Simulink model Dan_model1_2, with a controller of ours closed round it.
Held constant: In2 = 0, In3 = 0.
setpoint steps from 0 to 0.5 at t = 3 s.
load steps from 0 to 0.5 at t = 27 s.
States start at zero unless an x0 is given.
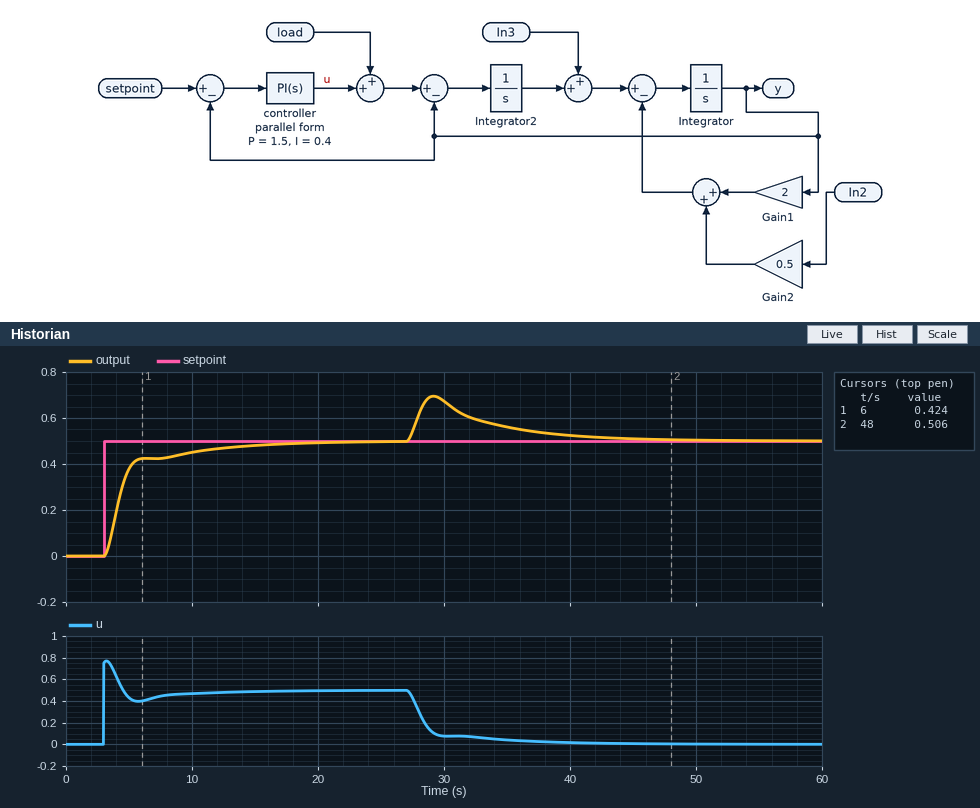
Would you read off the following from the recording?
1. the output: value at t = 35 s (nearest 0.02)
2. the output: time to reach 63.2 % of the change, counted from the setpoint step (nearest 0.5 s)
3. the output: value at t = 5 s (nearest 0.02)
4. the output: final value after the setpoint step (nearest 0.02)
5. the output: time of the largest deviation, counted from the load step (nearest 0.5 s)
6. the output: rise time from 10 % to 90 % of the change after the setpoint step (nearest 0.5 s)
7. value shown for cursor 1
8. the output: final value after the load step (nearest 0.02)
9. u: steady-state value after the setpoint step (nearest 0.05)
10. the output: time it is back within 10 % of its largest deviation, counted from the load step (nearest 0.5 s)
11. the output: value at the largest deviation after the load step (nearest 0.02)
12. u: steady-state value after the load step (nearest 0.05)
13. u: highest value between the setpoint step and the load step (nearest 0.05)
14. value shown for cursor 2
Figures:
0.56
1.5 s
0.38
0.50
2.0 s
6.5 s
0.424
0.50
0.50
14.0 s
0.70
0.00
0.75
0.506
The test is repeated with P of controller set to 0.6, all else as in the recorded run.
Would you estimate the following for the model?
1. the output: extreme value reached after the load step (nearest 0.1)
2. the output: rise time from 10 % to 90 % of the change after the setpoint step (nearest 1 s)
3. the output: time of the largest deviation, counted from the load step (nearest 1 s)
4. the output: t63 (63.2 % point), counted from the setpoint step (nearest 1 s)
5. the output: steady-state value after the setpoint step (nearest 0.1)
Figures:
0.8
4 s
3 s
3 s
0.5
